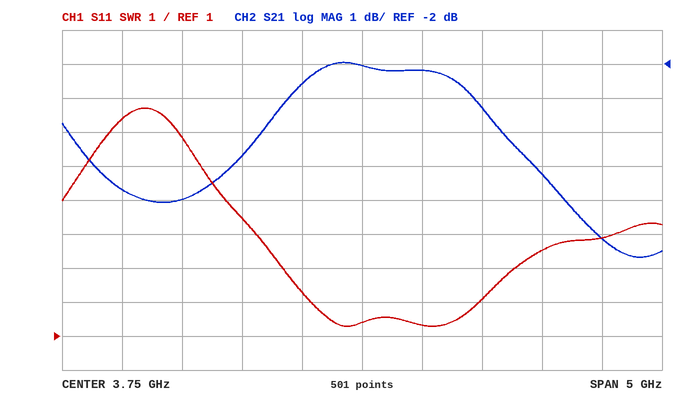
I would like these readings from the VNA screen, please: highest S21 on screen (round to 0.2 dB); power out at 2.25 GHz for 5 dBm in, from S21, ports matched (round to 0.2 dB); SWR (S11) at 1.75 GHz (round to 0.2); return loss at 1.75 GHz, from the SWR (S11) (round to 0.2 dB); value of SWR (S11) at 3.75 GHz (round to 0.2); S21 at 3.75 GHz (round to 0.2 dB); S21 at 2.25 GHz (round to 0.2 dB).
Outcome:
-2.0 dB
-1.0 dBm
7.4
2.4 dB
1.4
-2.0 dB
-6.0 dB
